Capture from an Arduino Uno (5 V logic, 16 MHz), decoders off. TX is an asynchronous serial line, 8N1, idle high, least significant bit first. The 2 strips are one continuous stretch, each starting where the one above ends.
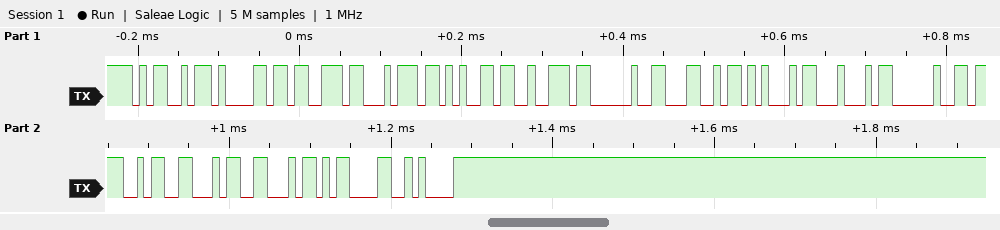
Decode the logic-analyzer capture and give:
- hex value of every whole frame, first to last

0x4D 0x61 0x73 0x74 0x65 0x72 0x20 0x4C 0x45 0x44 0x20 0x4F 0x46 0x46 0x0D 0x0A
